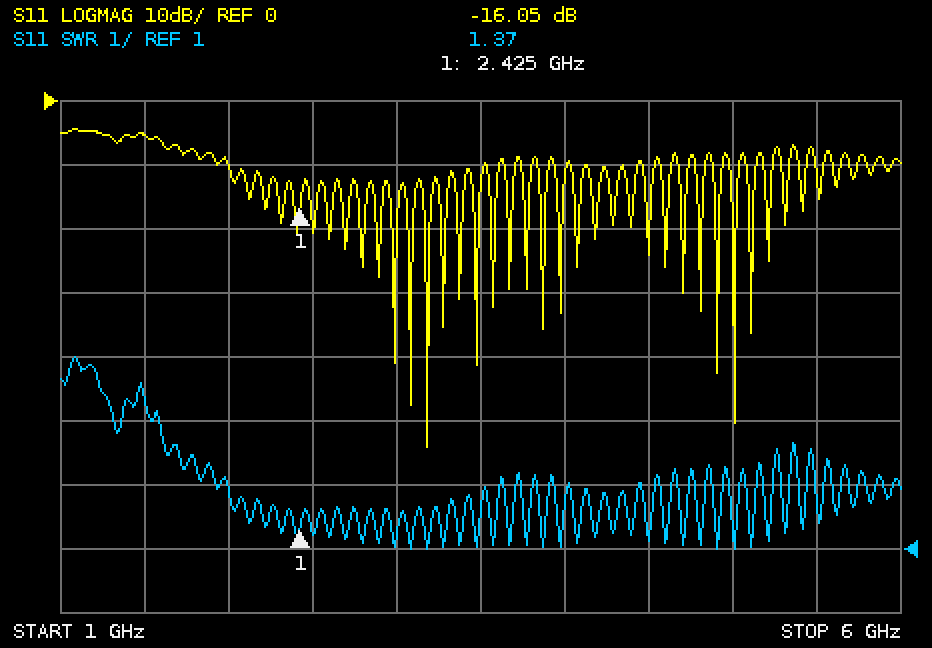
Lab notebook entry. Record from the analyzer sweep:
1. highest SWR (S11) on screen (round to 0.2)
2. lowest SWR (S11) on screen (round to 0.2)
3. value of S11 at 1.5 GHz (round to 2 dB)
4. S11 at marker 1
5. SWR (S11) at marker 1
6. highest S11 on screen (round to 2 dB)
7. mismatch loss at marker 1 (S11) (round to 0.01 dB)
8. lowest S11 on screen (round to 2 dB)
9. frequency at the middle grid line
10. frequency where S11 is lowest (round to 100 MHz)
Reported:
4.0
1.0
-6 dB
-16.05 dB
1.37
-4 dB
0.11 dB
-54 dB
3.5 GHz
3.2 GHz
